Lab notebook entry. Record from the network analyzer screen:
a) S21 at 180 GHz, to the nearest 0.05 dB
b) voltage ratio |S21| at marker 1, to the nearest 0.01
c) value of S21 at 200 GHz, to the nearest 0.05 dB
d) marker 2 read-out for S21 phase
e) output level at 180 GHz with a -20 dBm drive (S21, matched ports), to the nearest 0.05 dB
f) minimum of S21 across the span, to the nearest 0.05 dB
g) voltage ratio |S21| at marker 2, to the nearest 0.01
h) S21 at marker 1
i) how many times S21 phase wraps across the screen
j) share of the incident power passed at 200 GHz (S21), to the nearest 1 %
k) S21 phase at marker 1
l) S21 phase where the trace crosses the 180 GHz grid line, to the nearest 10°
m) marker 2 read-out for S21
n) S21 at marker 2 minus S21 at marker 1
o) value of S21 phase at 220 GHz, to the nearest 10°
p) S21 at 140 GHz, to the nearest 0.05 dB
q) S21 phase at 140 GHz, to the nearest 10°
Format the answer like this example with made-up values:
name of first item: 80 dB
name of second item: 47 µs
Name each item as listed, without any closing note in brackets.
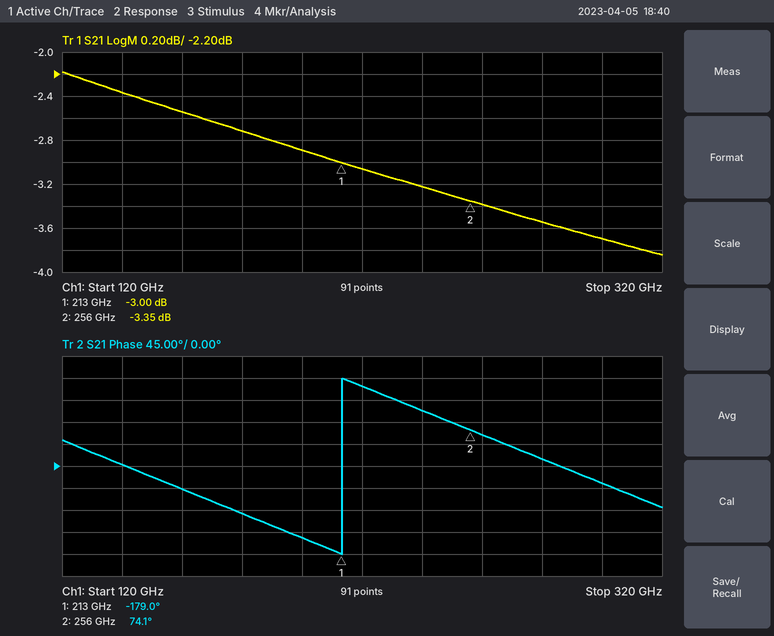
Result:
S21 at 180 GHz, to the nearest 0.05 dB: -2.70 dB
voltage ratio |S21| at marker 1, to the nearest 0.01: 0.71
value of S21 at 200 GHz, to the nearest 0.05 dB: -2.90 dB
marker 2 read-out for S21 phase: 74.1°
output level at 180 GHz with a -20 dBm drive (S21, matched ports), to the nearest 0.05 dB: -22.70 dBm
minimum of S21 across the span, to the nearest 0.05 dB: -3.85 dB
voltage ratio |S21| at marker 2, to the nearest 0.01: 0.68
S21 at marker 1: -3.00 dB
how many times S21 phase wraps across the screen: 1
share of the incident power passed at 200 GHz (S21), to the nearest 1 %: 51 %
S21 phase at marker 1: -179.0°
S21 phase where the trace crosses the 180 GHz grid line, to the nearest 10°: -100°
marker 2 read-out for S21: -3.35 dB
S21 at marker 2 minus S21 at marker 1: -0.35 dB
value of S21 phase at 220 GHz, to the nearest 10°: 160°
S21 at 140 GHz, to the nearest 0.05 dB: -2.35 dB
S21 phase at 140 GHz, to the nearest 10°: 0°
